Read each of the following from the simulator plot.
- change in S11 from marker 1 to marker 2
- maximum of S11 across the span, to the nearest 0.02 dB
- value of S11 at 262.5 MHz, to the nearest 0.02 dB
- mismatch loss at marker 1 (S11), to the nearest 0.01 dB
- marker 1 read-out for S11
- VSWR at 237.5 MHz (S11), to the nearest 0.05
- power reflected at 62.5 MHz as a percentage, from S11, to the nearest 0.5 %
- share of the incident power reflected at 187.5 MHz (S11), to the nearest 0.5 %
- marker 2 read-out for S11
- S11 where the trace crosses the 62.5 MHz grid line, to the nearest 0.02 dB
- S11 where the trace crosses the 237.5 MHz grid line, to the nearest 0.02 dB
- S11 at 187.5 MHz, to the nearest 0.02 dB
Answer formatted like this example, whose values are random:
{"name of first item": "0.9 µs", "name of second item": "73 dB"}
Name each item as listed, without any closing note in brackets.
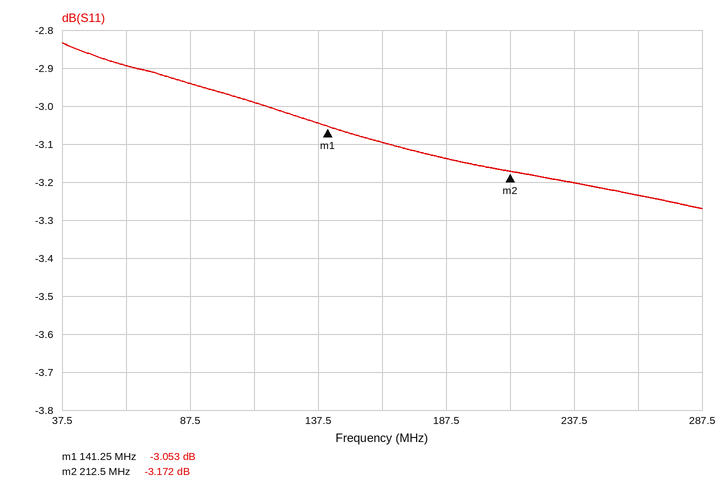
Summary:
{"change in S11 from marker 1 to marker 2": "-0.119 dB", "maximum of S11 across the span, to the nearest 0.02 dB": "-2.84 dB", "value of S11 at 262.5 MHz, to the nearest 0.02 dB": "-3.24 dB", "mismatch loss at marker 1 (S11), to the nearest 0.01 dB": "2.97 dB", "marker 1 read-out for S11": "-3.053 dB", "VSWR at 237.5 MHz (S11), to the nearest 0.05": "5.50", "power reflected at 62.5 MHz as a percentage, from S11, to the nearest 0.5 %": "51.5 %", "share of the incident power reflected at 187.5 MHz (S11), to the nearest 0.5 %": "48.5 %", "marker 2 read-out for S11": "-3.172 dB", "S11 where the trace crosses the 62.5 MHz grid line, to the nearest 0.02 dB": "-2.90 dB", "S11 where the trace crosses the 237.5 MHz grid line, to the nearest 0.02 dB": "-3.20 dB", "S11 at 187.5 MHz, to the nearest 0.02 dB": "-3.14 dB"}
